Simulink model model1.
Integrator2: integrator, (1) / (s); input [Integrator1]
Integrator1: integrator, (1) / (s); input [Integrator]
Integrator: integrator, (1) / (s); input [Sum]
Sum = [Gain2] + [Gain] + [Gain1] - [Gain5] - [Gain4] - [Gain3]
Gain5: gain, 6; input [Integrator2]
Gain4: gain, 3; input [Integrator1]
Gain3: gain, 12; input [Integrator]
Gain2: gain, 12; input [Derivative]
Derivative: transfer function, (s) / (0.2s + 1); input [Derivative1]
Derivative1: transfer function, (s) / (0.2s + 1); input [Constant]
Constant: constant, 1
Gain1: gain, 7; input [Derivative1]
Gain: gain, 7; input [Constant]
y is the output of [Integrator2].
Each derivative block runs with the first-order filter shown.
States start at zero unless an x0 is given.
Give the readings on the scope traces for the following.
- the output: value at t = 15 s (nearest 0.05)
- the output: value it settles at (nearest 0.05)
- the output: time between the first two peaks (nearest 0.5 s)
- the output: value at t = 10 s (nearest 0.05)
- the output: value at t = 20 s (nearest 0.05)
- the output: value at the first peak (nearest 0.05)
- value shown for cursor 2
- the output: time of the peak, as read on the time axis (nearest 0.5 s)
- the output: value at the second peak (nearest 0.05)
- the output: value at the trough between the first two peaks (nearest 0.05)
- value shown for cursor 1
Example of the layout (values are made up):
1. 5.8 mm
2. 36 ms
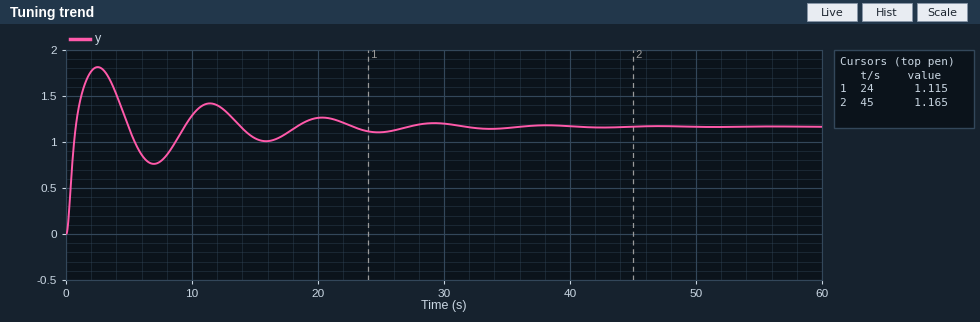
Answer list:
1. 1.05
2. 1.15
3. 9.0 s
4. 1.30
5. 1.25
6. 1.80
7. 1.165
8. 2.5 s
9. 1.40
10. 0.75
11. 1.115
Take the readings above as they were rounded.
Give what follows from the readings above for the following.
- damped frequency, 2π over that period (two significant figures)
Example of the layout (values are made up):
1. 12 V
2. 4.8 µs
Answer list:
1. 0.70 rad/s
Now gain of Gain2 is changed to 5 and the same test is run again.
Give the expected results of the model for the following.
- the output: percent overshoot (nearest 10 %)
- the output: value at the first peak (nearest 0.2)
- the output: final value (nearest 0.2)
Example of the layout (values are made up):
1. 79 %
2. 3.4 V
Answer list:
1. 70 %
2. 2.0
3. 1.2
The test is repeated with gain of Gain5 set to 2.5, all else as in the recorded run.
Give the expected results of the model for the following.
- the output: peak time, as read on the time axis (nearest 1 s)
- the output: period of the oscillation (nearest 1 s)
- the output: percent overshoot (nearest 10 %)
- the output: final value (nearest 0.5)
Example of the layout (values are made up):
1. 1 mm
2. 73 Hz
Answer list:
1. 6 s
2. 14 s
3. 30 %
4. 3.0
